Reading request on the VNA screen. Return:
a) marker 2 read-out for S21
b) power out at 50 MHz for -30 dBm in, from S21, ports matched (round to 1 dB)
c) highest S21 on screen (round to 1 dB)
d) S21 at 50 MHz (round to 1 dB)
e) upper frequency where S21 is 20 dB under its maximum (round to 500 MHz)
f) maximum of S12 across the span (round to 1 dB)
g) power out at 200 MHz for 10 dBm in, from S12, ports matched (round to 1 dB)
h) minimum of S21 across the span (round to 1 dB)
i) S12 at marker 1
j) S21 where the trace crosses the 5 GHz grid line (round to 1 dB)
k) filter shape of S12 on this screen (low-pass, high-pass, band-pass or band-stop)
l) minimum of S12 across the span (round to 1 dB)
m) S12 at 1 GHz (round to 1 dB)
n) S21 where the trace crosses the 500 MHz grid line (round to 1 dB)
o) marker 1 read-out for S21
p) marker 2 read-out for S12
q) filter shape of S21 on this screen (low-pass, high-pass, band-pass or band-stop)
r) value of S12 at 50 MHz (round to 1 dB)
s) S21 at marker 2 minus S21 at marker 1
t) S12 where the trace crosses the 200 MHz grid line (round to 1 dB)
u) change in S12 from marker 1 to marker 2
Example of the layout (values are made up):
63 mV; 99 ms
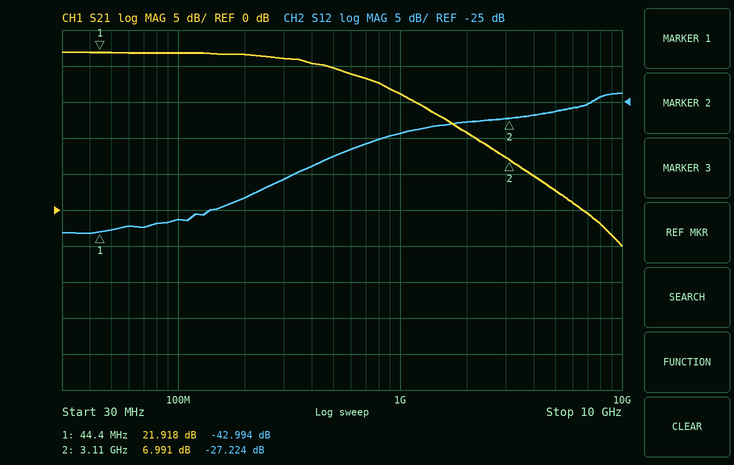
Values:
6.991 dB; -8 dBm; 22 dB; 22 dB; 5.5 GHz; -24 dB; -28 dBm; -5 dB; -42.994 dB; 3 dB; high-pass; -43 dB; -29 dB; 20 dB; 21.918 dB; -27.224 dB; low-pass; -43 dB; -14.927 dB; -38 dB; 15.770 dB
